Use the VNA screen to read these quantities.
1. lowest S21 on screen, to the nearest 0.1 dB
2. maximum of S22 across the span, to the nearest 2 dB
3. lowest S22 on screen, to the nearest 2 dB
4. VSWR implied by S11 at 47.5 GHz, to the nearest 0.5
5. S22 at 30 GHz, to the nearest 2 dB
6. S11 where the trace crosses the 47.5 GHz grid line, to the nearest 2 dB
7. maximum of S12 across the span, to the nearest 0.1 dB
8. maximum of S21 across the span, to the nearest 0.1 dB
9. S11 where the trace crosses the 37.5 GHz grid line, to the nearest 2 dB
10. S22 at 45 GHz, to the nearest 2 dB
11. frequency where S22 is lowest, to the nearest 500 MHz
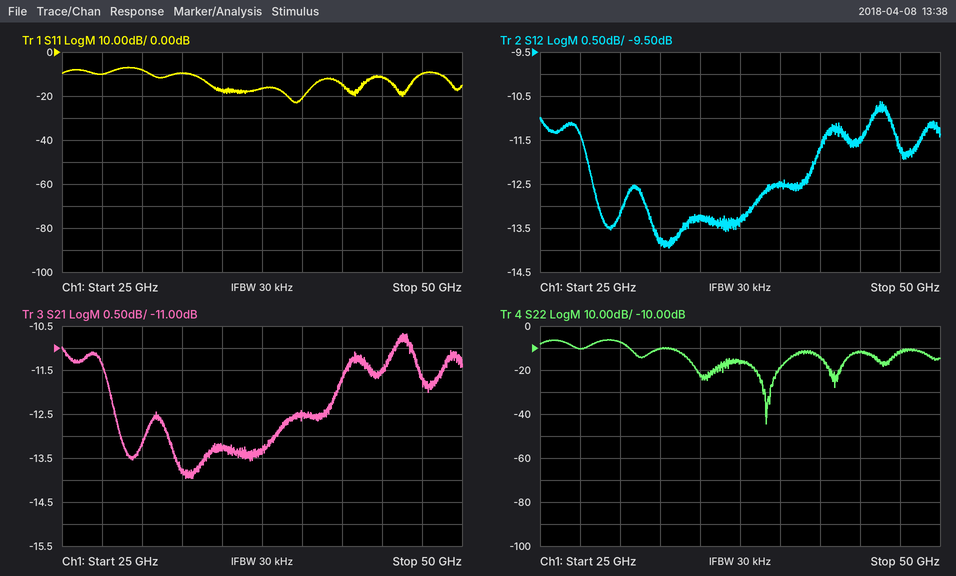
-14.0 dB
-6 dB
-44 dB
2.0
-8 dB
-10 dB
-10.6 dB
-10.7 dB
-16 dB
-12 dB
39.0 GHz
